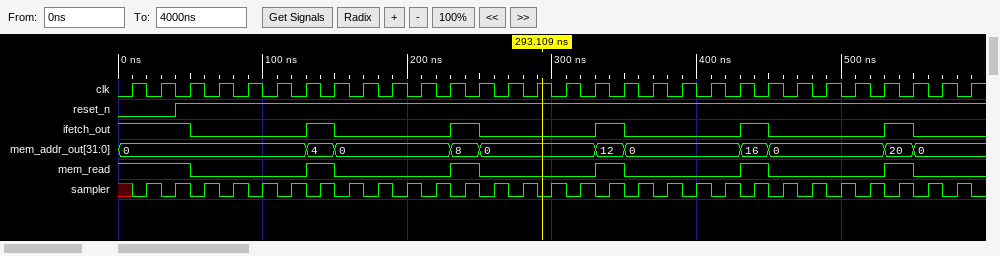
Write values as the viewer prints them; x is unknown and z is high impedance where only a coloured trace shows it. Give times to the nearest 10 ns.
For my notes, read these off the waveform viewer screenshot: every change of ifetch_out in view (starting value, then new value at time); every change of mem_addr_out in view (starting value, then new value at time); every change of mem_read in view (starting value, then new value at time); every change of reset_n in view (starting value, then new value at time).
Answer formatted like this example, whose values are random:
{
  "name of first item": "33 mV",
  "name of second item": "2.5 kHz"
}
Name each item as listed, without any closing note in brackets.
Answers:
{
  "every change of ifetch_out in view": "1, 0 at 50 ns, 1 at 130 ns, 0 at 150 ns, 1 at 230 ns, 0 at 250 ns, 1 at 330 ns, 0 at 350 ns, 1 at 430 ns, 0 at 450 ns, 1 at 530 ns, 0 at 550 ns",
  "every change of mem_addr_out in view": "0, 4 at 130 ns, 0 at 150 ns, 8 at 230 ns, 0 at 250 ns, 12 at 330 ns, 0 at 350 ns, 16 at 430 ns, 0 at 450 ns, 20 at 530 ns, 0 at 550 ns",
  "every change of mem_read in view": "1, 0 at 50 ns, 1 at 130 ns, 0 at 150 ns, 1 at 230 ns, 0 at 250 ns, 1 at 330 ns, 0 at 350 ns, 1 at 430 ns, 0 at 450 ns, 1 at 530 ns, 0 at 550 ns",
  "every change of reset_n in view": "0, 1 at 40 ns"
}
